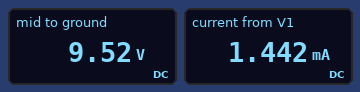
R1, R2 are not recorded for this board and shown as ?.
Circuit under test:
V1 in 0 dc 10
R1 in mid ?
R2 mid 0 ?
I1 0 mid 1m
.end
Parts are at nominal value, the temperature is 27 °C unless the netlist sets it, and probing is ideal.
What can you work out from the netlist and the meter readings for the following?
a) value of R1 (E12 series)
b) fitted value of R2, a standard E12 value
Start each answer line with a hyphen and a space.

- 330 Ω
- 3.9 kΩ
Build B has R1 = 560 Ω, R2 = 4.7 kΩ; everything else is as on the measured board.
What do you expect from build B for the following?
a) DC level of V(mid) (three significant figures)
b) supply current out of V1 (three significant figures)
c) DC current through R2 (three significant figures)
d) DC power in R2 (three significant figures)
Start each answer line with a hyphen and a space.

- 9.44 V
- 1.01 mA
- 2.01 mA
- 18.9 mW
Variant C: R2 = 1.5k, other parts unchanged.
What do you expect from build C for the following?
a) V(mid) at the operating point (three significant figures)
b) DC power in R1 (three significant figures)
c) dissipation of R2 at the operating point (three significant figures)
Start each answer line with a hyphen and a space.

- 8.47 V
- 7.12 mW
- 47.8 mW
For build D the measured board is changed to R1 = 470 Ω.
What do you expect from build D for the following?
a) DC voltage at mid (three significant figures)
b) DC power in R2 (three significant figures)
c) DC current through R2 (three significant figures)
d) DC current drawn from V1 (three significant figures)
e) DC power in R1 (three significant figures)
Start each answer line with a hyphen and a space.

- 9.34 V
- 22.4 mW
- 2.40 mA
- 1.40 mA
- 916 µW
